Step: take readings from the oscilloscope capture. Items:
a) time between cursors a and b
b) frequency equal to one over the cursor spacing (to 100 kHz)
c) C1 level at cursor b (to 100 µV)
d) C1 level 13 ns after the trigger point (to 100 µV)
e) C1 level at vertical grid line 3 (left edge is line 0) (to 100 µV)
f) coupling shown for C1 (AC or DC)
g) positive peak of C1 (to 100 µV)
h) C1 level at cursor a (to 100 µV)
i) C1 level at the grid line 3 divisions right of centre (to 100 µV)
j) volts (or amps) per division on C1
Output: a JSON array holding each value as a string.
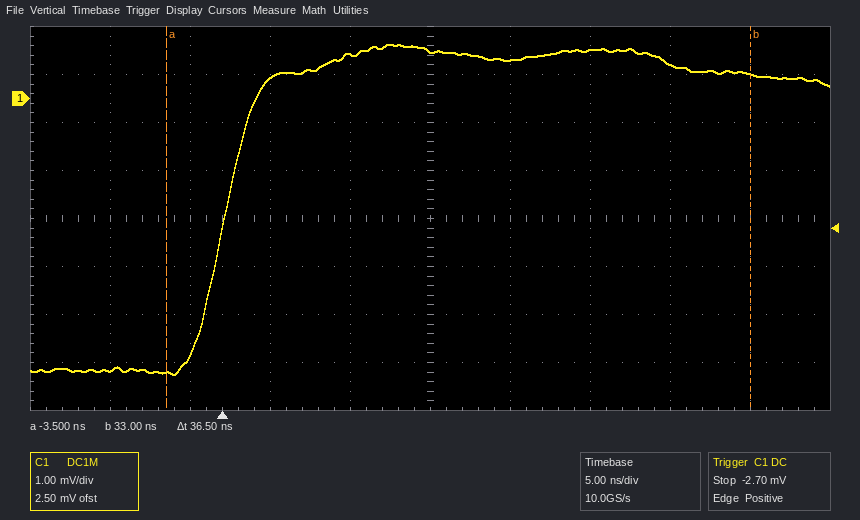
["36.5 ns", "27.4 MHz", "500 µV", "1.0 mV", "400 µV", "DC", "1.1 mV", "-5.7 mV", "700 µV", "1 mV"]
